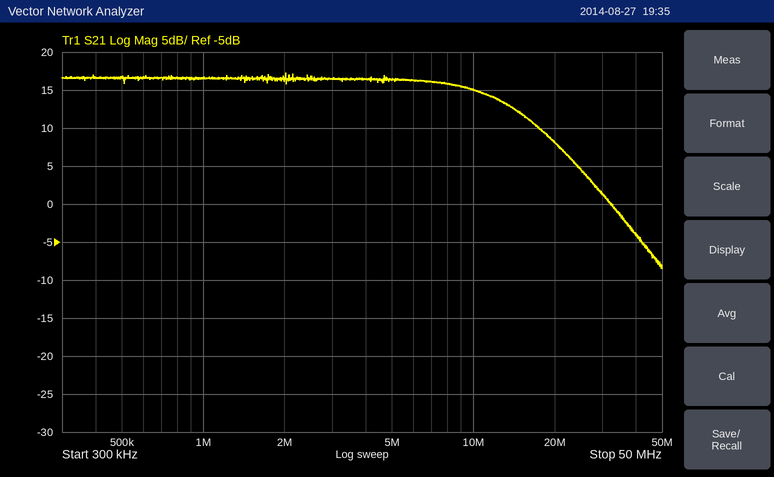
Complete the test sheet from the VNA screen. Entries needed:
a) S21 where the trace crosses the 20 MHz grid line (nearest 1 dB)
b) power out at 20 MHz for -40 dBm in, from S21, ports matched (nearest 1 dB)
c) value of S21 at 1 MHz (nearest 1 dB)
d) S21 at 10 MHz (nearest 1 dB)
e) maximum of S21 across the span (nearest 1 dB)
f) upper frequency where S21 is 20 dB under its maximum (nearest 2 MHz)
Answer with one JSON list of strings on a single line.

["8 dB", "-32 dBm", "17 dB", "15 dB", "17 dB", "38 MHz"]
